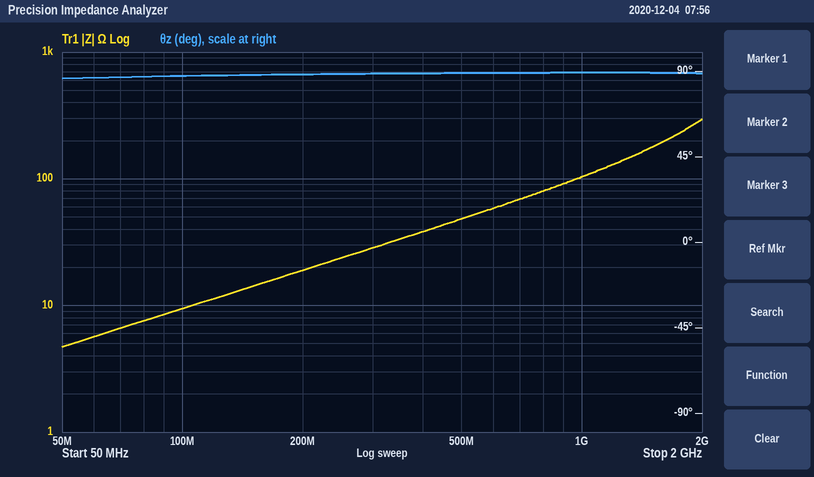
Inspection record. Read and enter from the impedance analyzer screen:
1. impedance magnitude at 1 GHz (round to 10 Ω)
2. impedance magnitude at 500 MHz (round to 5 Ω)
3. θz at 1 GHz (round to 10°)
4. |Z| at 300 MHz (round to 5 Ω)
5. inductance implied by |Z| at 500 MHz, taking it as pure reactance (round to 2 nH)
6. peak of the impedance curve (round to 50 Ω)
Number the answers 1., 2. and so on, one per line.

1. 100 Ω
2. 50 Ω
3. 90°
4. 30 Ω
5. 16 nH
6. 300 Ω
